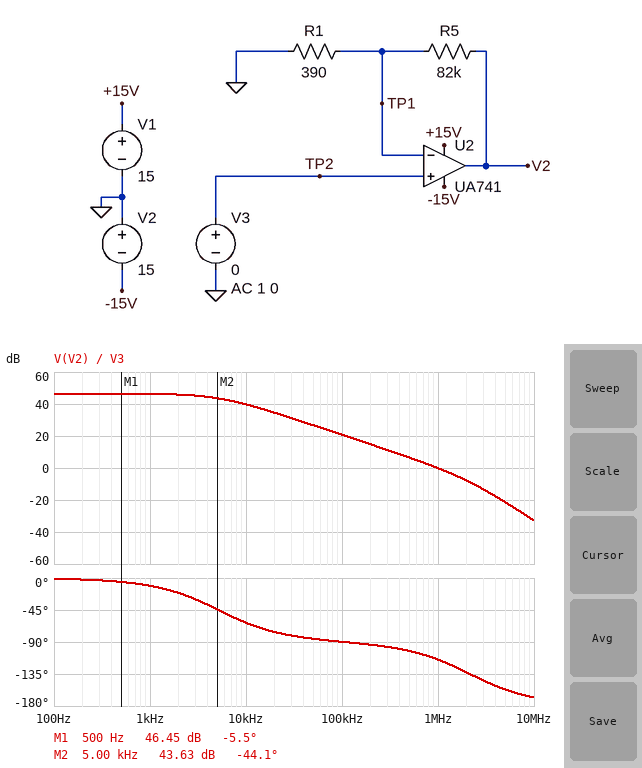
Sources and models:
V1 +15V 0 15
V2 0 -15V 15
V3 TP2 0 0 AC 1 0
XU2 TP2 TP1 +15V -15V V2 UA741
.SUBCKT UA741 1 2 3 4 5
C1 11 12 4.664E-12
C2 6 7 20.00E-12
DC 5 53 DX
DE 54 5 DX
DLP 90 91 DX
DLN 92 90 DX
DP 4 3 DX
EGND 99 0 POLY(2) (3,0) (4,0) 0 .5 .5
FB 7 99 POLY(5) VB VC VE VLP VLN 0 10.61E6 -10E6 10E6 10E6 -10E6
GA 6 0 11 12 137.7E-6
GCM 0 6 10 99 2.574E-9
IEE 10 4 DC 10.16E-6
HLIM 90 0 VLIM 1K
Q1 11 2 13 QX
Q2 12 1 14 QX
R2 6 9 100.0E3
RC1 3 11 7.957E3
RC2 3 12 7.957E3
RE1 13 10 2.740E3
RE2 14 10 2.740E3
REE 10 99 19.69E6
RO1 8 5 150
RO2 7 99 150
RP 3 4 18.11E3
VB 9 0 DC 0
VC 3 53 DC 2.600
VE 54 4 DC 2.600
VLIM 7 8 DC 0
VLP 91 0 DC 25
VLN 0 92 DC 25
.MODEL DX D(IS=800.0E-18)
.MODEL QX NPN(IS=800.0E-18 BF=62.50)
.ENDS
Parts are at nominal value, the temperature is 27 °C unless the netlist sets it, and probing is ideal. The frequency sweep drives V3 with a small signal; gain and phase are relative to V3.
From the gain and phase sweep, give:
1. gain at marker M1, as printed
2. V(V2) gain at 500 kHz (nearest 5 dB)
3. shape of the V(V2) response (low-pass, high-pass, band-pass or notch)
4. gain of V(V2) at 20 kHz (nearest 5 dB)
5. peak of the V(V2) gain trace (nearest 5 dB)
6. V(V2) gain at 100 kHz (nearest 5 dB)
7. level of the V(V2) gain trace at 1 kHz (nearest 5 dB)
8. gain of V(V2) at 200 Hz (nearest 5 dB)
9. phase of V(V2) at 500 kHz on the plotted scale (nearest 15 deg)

46.45 dB
5 dB
low-pass
35 dB
45 dB
20 dB
45 dB
45 dB
-105 deg
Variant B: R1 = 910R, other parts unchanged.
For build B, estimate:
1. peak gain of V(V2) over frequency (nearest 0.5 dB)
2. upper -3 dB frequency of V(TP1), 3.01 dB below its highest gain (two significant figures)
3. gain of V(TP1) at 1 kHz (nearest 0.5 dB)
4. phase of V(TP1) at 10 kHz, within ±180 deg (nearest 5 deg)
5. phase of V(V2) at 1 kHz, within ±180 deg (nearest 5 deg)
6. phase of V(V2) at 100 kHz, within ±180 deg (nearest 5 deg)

39.0 dB
12 kHz
0 dB
-40 deg
-5 deg
-85 deg
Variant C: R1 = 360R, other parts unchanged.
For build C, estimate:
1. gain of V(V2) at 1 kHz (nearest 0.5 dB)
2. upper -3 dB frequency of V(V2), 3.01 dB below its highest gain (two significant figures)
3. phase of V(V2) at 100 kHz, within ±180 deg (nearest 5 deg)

47.0 dB
4.8 kHz
-90 deg
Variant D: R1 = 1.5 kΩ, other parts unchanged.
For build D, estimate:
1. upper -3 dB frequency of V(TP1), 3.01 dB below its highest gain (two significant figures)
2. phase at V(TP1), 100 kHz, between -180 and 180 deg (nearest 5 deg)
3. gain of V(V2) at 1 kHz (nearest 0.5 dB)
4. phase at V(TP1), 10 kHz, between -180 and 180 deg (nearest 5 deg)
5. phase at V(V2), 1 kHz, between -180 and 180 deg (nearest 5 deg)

20 kHz
-80 deg
35.0 dB
-25 deg
-5 deg
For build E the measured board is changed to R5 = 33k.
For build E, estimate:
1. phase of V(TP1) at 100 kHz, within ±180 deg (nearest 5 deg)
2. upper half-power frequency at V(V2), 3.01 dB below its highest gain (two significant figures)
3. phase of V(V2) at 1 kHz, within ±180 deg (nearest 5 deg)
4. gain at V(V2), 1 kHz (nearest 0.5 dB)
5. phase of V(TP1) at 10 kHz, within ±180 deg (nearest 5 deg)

-85 deg
13 kHz
-5 deg
38.5 dB
-40 deg
